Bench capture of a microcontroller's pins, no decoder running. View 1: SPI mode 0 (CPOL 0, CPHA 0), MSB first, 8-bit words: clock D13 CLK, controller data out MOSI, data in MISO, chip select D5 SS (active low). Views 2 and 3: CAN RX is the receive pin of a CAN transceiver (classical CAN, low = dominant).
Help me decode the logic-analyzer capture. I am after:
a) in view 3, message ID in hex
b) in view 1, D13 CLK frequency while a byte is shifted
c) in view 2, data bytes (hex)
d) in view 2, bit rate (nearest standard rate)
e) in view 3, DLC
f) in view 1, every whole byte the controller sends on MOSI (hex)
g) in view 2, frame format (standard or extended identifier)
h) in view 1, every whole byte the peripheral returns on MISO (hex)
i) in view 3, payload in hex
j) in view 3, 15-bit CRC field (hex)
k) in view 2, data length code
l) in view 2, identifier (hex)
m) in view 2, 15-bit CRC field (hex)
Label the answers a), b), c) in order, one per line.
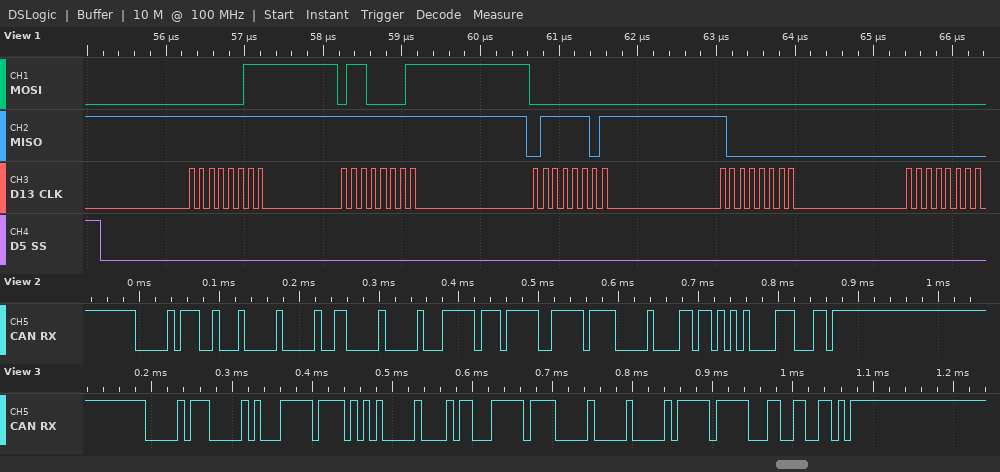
a) 0x038
b) 8 MHz
c) 00 60 00 FF 7D FF 00 6D
d) 125 kbit/s
e) 8
f) 03 61 00 00 00
g) standard
h) FF FF 7D 80 00
i) FF AA 00 B1 FF 00 00 FF
j) 0x6666
k) 8
l) 0x039
m) 0x2871
